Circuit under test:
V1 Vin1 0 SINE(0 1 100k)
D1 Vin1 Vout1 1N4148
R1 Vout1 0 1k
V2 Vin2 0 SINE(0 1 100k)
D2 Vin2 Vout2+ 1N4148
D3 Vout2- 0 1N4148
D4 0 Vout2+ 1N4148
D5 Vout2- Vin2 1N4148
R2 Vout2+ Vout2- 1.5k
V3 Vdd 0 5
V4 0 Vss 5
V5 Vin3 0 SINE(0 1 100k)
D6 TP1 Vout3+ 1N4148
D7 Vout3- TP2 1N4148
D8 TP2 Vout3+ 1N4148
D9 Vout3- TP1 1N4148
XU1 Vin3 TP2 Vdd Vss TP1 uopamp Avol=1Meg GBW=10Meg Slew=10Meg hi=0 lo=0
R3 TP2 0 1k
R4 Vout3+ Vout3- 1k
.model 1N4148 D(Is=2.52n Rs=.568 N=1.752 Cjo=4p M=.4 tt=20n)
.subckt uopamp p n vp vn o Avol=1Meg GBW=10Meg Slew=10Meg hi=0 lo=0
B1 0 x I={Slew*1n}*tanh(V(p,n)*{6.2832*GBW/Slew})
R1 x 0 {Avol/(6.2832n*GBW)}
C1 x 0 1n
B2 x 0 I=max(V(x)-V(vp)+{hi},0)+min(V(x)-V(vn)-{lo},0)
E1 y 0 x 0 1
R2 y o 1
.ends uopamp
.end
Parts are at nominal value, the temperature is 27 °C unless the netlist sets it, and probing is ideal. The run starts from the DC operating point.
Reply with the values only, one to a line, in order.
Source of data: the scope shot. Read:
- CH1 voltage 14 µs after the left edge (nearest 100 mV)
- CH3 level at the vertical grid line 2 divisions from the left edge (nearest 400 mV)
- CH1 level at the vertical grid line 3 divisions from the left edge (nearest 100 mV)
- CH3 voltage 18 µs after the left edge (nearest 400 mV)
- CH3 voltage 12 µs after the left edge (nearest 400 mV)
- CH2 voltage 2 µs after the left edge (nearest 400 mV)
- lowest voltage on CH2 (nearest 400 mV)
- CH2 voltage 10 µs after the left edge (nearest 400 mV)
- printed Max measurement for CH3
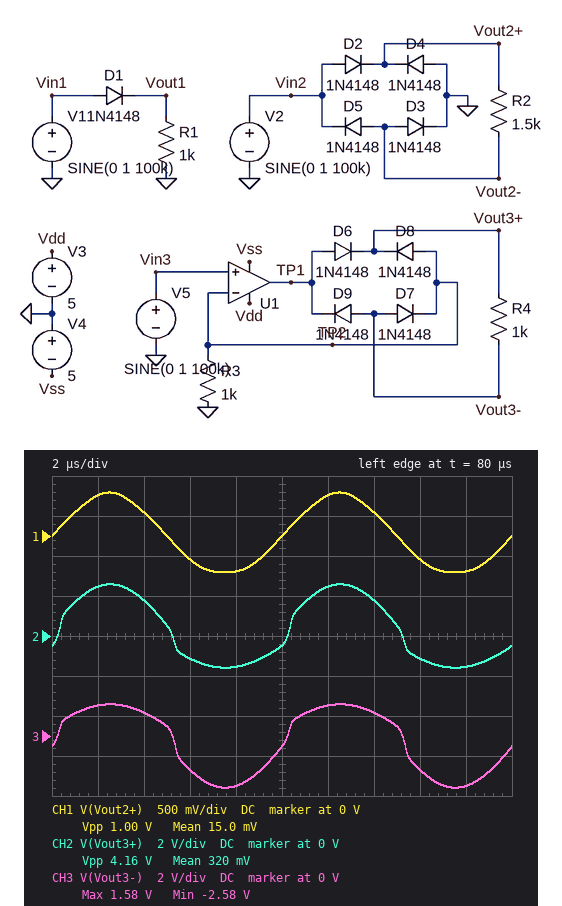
300 mV
1.2 V
-300 mV
-2.4 V
1.6 V
2.4 V
-1.6 V
-400 mV
1.58 V
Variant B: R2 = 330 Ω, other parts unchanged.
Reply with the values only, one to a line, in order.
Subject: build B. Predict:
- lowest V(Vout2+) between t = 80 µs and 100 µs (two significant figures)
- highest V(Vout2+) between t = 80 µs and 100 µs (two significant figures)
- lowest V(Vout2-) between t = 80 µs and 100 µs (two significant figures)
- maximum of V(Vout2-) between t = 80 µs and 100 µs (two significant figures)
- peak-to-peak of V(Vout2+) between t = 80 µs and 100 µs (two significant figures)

-480 mV
520 mV
-520 mV
480 mV
1.0 V
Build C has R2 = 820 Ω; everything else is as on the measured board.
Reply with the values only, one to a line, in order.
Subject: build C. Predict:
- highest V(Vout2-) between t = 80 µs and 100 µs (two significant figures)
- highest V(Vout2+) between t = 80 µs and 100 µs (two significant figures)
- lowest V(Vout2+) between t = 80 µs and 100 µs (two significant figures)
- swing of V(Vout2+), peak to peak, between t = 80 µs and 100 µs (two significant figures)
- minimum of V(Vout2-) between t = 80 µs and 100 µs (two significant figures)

470 mV
530 mV
-470 mV
1.0 V
-530 mV
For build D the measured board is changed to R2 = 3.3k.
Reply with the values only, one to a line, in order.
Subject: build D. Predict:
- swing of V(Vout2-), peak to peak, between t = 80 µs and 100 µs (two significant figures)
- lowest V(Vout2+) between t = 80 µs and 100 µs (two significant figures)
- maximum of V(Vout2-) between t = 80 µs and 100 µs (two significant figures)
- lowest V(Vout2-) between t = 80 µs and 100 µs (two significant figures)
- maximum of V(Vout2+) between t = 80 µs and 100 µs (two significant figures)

1.0 V
-440 mV
440 mV
-560 mV
560 mV
